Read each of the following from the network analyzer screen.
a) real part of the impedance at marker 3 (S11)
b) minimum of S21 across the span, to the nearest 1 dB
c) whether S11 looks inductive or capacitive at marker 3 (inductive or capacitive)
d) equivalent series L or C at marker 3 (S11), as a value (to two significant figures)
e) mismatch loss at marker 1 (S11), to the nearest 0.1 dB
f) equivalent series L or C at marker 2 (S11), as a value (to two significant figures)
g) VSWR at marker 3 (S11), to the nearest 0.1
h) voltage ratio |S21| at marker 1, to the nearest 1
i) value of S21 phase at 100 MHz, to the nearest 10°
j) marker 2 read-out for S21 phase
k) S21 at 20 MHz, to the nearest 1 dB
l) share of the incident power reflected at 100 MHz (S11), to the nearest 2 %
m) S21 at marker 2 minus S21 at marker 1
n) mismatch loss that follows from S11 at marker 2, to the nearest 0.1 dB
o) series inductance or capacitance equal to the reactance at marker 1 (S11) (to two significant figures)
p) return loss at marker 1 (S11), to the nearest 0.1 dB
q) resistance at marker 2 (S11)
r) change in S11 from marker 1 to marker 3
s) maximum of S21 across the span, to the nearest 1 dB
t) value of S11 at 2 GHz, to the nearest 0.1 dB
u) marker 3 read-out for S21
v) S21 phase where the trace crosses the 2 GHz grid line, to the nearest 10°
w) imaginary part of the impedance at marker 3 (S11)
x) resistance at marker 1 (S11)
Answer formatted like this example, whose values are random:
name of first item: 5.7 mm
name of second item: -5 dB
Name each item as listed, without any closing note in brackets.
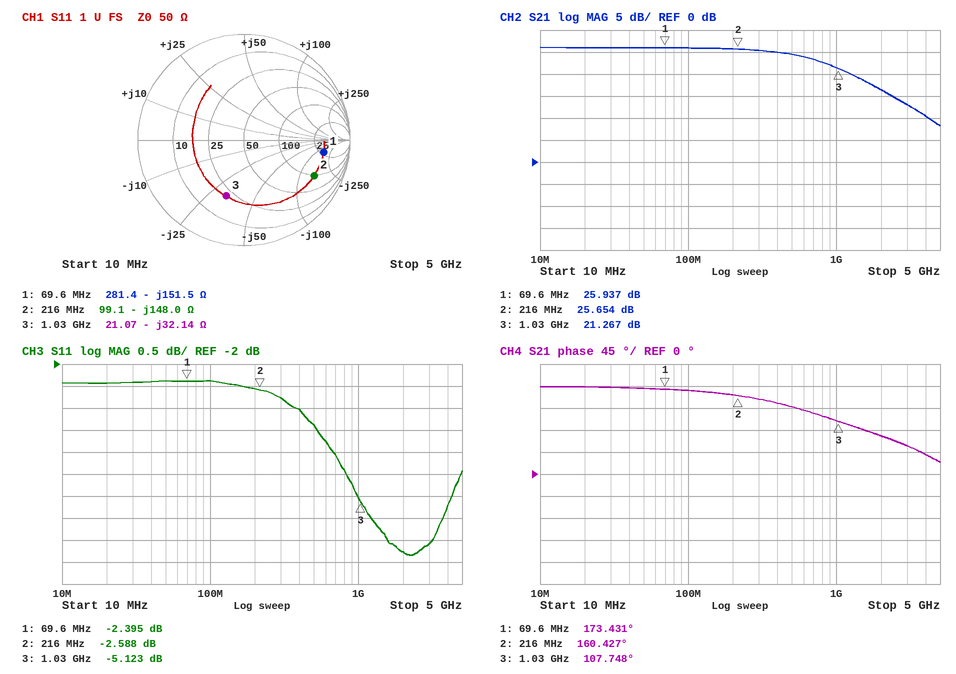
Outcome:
real part of the impedance at marker 3: 21.07 Ω
minimum of S21 across the span, to the nearest 1 dB: 8 dB
whether S11 looks inductive or capacitive at marker 3: capacitive
equivalent series L or C at marker 3 (S11), as a value: 4.8 pF
mismatch loss at marker 1 (S11), to the nearest 0.1 dB: 3.7 dB
equivalent series L or C at marker 2 (S11), as a value: 5.0 pF
VSWR at marker 3 (S11), to the nearest 0.1: 3.5
voltage ratio |S21| at marker 1, to the nearest 1: 20
value of S21 phase at 100 MHz, to the nearest 10°: 170°
marker 2 read-out for S21 phase: 160.427°
S21 at 20 MHz, to the nearest 1 dB: 26 dB
share of the incident power reflected at 100 MHz (S11), to the nearest 2 %: 58 %
S21 at marker 2 minus S21 at marker 1: -0.283 dB
mismatch loss that follows from S11 at marker 2, to the nearest 0.1 dB: 3.5 dB
series inductance or capacitance equal to the reactance at marker 1 (S11): 15 pF
return loss at marker 1 (S11), to the nearest 0.1 dB: 2.4 dB
resistance at marker 2: 99.1 Ω
change in S11 from marker 1 to marker 3: -2.728 dB
maximum of S21 across the span, to the nearest 1 dB: 26 dB
value of S11 at 2 GHz, to the nearest 0.1 dB: -6.3 dB
marker 3 read-out for S21: 21.267 dB
S21 phase where the trace crosses the 2 GHz grid line, to the nearest 10°: 80°
imaginary part of the impedance at marker 3: -32.14 Ω
resistance at marker 1: 281.4 Ω
